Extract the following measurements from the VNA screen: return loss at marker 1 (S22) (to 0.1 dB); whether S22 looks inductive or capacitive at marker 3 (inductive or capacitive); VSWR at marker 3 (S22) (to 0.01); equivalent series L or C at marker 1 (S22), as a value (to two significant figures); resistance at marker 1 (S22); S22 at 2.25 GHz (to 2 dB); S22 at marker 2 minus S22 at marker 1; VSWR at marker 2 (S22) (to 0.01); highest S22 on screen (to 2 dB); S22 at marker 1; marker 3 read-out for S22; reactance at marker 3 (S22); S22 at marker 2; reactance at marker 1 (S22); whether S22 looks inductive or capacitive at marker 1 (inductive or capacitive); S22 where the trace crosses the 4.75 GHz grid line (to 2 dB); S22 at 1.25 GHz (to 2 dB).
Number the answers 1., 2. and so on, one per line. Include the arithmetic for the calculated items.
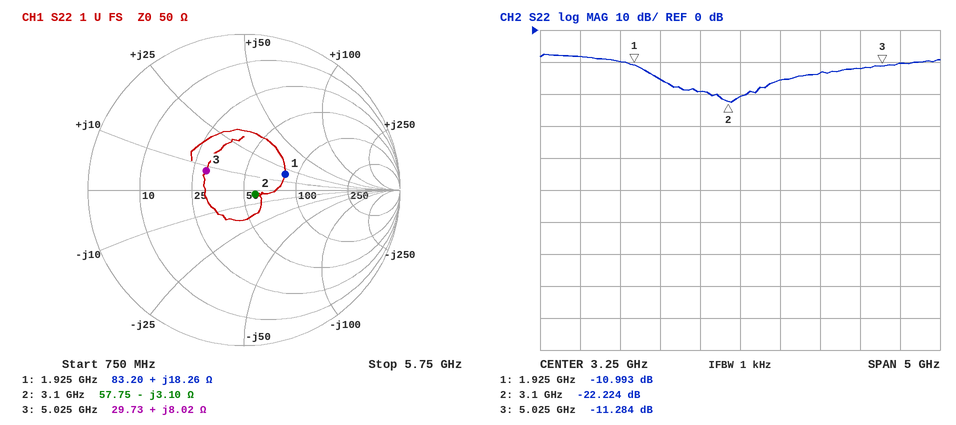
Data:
1. 11.0 dB
2. inductive
3. 1.75
4. L = 18.26 Ω/(2π × 1.925 GHz) ≈ 1.5 nH
5. 83.20 Ω
6. -16 dB
7. -22.224 − (-10.993) = -11.231 dB
8. 1.17
9. -8 dB
10. -10.993 dB
11. -11.284 dB
12. +8.02 Ω
13. -22.224 dB
14. +18.26 Ω
15. inductive
16. -12 dB
17. -8 dB
